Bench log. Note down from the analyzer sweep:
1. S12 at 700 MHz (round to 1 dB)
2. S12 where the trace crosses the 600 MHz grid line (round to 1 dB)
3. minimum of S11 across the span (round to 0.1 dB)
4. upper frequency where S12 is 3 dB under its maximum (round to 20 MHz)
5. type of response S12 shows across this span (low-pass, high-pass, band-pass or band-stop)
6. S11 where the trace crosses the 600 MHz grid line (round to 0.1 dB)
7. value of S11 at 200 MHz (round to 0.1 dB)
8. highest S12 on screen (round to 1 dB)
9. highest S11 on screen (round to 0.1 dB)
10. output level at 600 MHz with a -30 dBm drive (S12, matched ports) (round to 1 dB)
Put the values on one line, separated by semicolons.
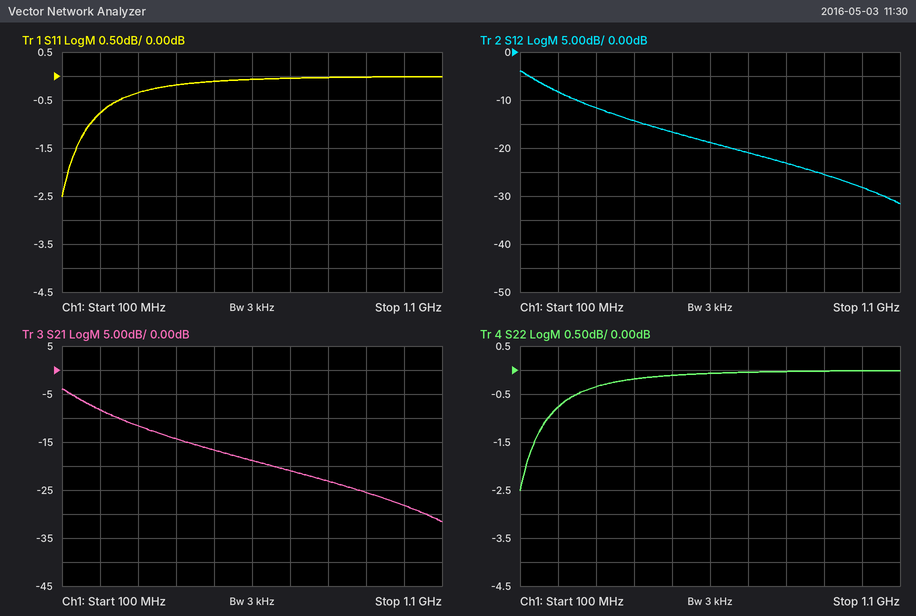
-21 dB; -19 dB; -2.5 dB; 160 MHz; low-pass; -0.1 dB; -0.8 dB; -4 dB; 0.0 dB; -49 dBm
